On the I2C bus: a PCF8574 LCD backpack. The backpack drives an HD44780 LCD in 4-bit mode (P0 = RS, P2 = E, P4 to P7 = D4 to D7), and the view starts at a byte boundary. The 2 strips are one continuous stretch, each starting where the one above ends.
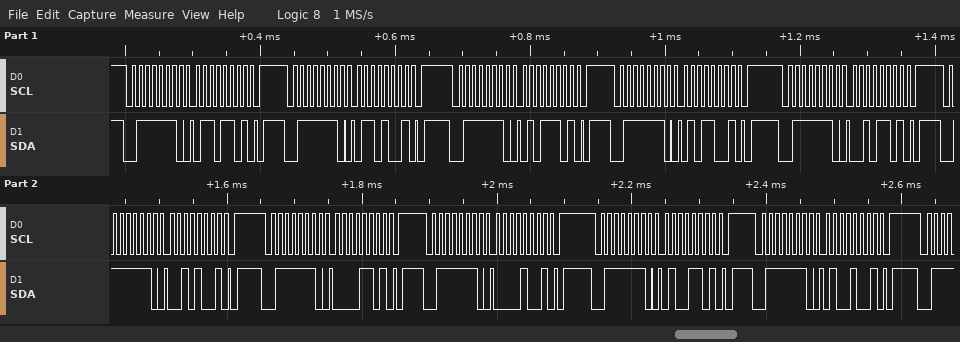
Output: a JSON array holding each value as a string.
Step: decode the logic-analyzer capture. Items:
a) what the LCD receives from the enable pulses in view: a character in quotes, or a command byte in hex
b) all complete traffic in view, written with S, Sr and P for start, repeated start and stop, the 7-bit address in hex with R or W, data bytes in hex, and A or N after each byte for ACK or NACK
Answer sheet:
["'e' ' '", "S 3FW A 6D A P S 3FW A 69 A P S 3FW A 5D A P S 3FW A 59 A P S 3FW A 2D A P S 3FW A 29 A P S 3FW A 0D A P S 3FW A 09 A P S 3FW A 4D A P S 3FW A 49 A P"]
